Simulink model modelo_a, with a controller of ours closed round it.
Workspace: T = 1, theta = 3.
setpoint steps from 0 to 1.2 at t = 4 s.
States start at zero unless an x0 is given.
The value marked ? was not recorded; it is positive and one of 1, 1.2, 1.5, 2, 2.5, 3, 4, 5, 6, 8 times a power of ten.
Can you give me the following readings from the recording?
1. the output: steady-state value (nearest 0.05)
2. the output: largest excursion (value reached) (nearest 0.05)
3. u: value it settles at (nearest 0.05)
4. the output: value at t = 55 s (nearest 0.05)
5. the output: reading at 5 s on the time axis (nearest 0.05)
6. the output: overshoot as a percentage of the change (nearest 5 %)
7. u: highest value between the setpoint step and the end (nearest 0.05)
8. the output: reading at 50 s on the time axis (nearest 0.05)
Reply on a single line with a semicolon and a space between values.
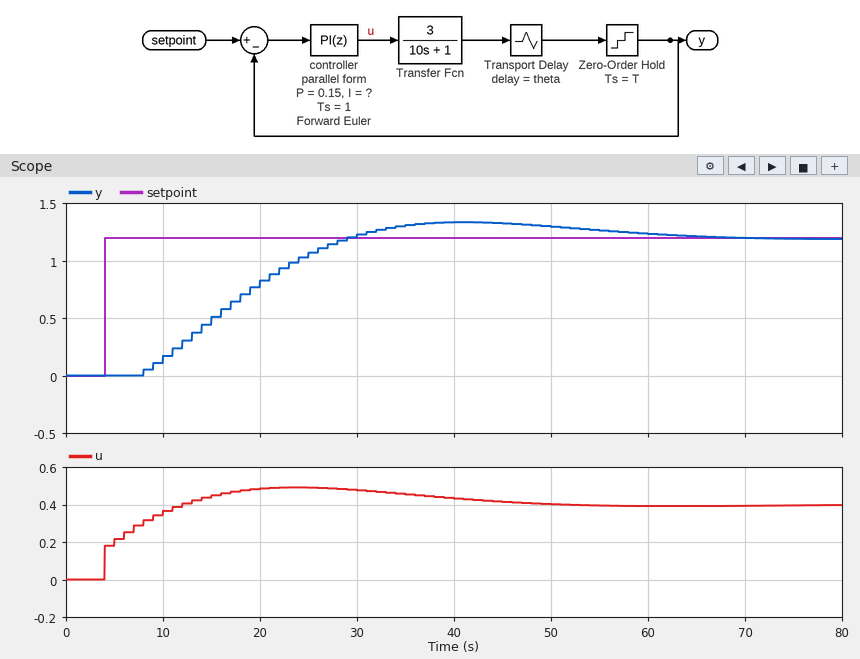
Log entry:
1.20; 1.35; 0.40; 1.25; 0.00; 10 %; 0.50; 1.30
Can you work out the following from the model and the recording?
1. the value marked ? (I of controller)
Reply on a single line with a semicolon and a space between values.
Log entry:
0.03
